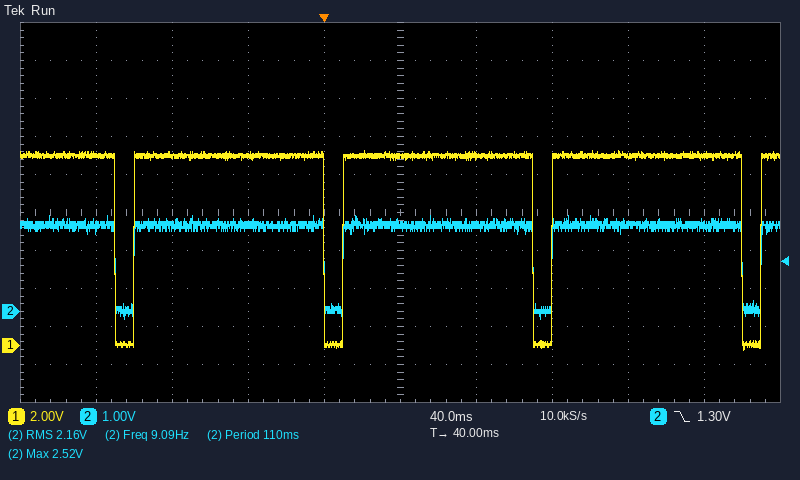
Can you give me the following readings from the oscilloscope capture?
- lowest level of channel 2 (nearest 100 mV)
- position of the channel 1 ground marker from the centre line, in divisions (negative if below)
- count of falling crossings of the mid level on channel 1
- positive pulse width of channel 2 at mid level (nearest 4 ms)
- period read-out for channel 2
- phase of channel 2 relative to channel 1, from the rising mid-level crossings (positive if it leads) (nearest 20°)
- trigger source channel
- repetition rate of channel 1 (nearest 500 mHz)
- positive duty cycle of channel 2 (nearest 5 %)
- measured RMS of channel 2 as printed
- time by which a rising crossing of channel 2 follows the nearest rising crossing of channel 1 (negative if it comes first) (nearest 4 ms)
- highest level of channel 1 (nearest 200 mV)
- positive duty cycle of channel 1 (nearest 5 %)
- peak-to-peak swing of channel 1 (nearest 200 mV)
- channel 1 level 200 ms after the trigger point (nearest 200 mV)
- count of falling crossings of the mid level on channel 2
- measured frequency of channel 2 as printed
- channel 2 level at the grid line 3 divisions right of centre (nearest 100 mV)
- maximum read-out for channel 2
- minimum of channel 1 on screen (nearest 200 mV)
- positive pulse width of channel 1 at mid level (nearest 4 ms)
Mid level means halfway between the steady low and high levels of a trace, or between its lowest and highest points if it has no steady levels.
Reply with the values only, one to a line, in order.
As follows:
-200 mV
-3.5 div
4
100 ms
110 ms
0°
channel 2
9.0 Hz
90 %
2.16 V
0 ms
10.2 V
90 %
10.4 V
10.0 V
4
9.09 Hz
2.3 V
2.52 V
-200 mV
100 ms
